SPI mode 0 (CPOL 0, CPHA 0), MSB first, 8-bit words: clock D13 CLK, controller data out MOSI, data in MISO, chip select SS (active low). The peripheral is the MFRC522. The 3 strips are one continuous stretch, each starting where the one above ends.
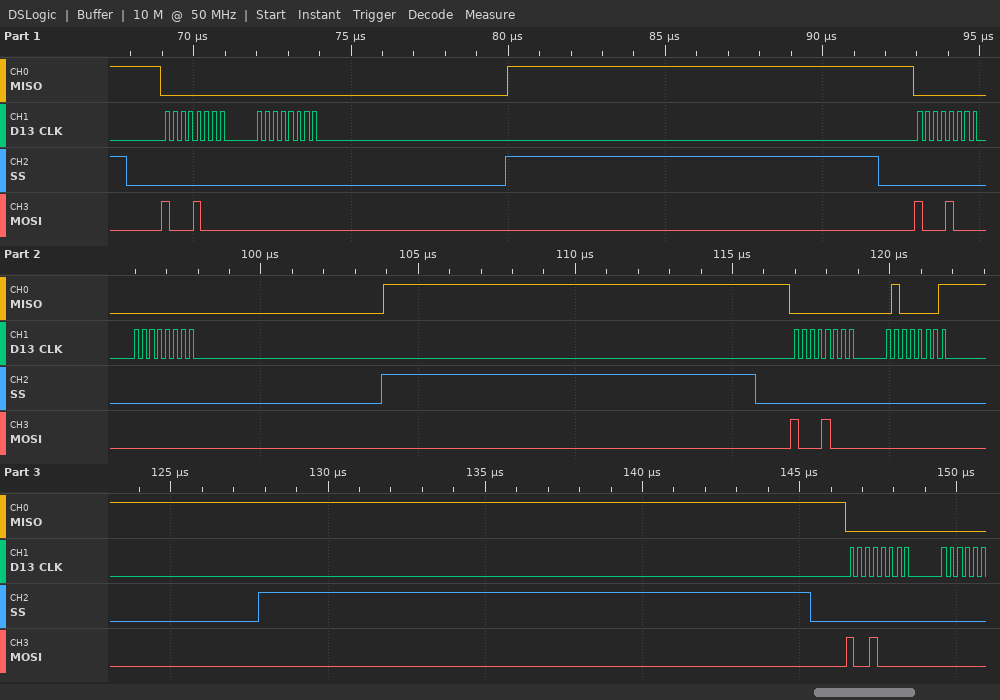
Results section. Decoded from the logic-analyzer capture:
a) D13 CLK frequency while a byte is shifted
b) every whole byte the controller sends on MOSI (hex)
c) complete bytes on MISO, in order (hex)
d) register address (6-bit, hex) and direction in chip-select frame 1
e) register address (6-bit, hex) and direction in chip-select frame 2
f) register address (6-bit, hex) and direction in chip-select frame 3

4 MHz
0x88 0x00 0x88 0x00 0x88 0x00 0x90
0x00 0x00 0x00 0x00 0x00 0x41 0x00
0x04 read
0x04 read
0x04 read
